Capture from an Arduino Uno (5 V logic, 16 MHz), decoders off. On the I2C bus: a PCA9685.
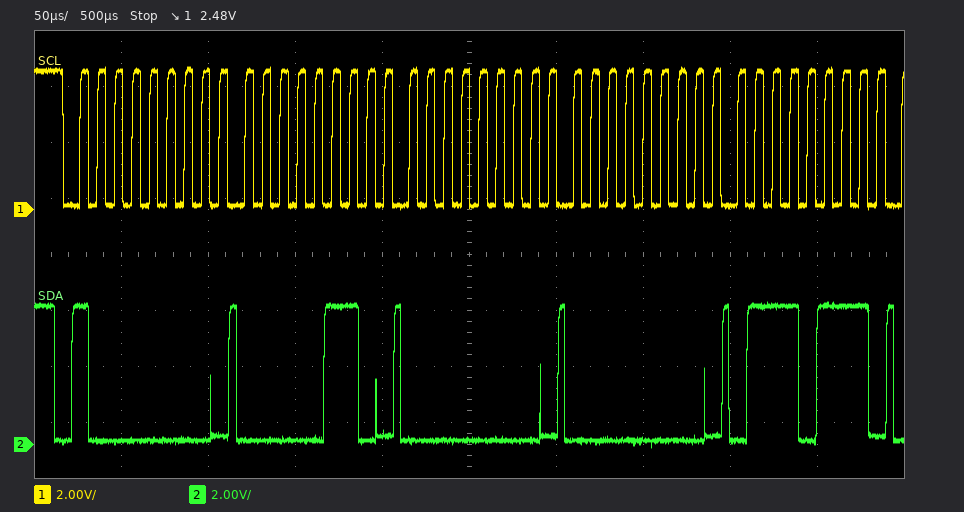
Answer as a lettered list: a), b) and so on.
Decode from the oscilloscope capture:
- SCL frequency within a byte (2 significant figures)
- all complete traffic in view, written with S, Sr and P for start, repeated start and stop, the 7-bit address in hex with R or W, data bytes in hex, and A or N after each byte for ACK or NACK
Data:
a) 100 kHz
b) S 40W A 06 A 00 A 00 A 77 A
